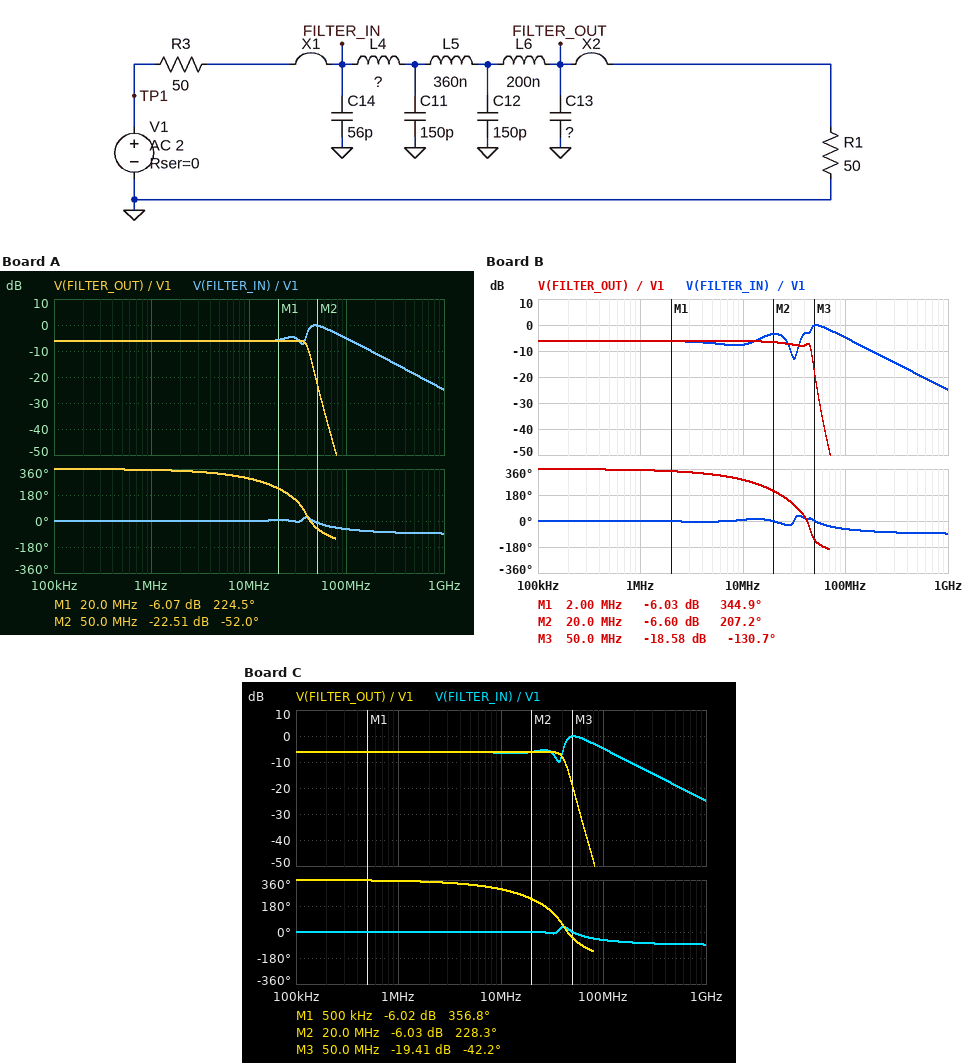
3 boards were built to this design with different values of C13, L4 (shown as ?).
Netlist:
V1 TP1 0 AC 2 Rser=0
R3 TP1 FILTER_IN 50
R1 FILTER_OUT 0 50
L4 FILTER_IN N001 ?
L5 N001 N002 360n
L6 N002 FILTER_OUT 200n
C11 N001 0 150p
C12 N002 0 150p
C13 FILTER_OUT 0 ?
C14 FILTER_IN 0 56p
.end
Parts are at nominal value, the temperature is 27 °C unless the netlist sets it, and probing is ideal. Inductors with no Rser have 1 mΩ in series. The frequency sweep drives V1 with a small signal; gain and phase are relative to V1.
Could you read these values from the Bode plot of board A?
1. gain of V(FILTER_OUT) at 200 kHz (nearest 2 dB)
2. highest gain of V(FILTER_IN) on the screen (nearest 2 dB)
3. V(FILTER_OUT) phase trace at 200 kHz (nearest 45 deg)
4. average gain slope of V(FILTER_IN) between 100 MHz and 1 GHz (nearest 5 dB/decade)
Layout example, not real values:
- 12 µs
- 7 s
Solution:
- -6 dB
- 0 dB
- 360 deg
- -20 dB/decade
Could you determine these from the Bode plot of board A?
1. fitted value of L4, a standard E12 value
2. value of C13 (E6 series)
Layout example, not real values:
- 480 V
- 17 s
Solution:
- 330 nH
- 15 pF
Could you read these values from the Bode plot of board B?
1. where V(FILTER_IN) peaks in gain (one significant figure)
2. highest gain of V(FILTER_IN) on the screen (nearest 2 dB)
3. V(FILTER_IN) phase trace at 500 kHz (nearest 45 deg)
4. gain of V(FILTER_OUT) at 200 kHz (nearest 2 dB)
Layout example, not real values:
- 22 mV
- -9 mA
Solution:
- 50 MHz
- 0 dB
- 0 deg
- -6 dB
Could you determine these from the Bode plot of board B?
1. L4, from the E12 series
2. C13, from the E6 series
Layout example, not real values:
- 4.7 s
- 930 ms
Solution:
- 270 nH
- 150 pF
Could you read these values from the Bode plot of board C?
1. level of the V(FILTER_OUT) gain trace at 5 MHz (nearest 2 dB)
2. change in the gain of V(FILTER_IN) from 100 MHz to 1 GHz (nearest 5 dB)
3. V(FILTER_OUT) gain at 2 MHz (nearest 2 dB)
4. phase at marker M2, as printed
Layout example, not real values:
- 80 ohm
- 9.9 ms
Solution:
- -6 dB
- -20 dB
- -6 dB
- 228.3 deg
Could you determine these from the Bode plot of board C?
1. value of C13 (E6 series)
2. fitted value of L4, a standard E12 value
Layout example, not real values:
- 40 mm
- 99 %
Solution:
- 22 pF
- 270 nH
